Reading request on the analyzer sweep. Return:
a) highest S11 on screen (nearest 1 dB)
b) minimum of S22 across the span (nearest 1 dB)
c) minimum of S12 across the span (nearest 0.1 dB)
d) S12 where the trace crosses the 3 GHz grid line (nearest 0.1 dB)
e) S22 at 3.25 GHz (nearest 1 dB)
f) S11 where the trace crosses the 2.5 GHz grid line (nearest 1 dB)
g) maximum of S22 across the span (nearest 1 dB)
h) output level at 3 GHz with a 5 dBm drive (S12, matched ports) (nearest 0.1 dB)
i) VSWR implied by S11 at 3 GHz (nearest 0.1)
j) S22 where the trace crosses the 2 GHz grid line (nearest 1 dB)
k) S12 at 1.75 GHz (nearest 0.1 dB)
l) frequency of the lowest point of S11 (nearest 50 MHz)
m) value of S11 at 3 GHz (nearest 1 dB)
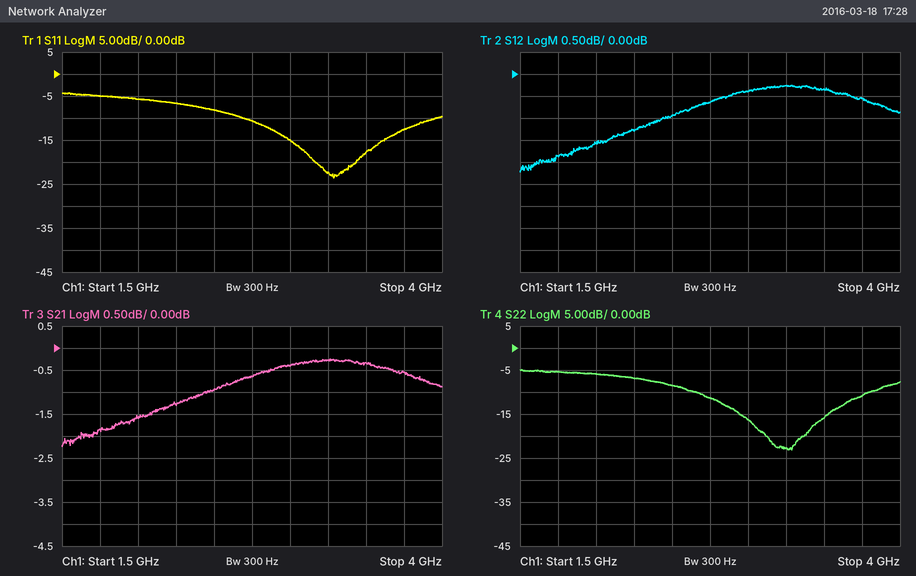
-4 dB
-23 dB
-2.2 dB
-0.4 dB
-23 dB
-8 dB
-5 dB
4.6 dBm
1.4
-6 dB
-1.9 dB
3.30 GHz
-15 dB
